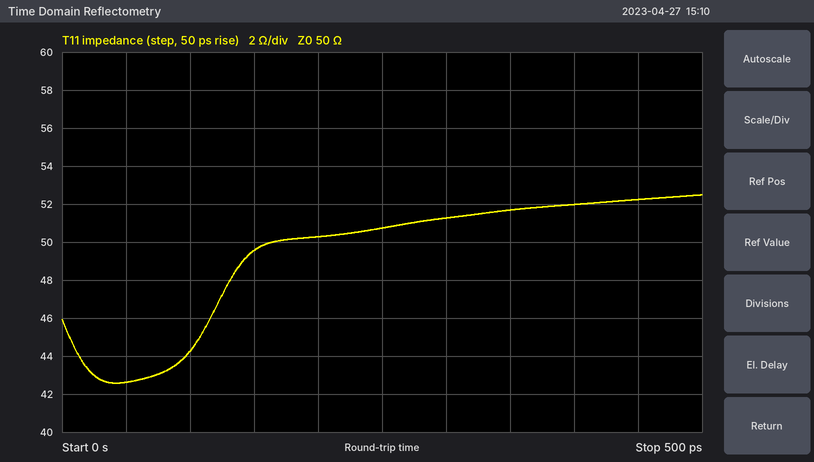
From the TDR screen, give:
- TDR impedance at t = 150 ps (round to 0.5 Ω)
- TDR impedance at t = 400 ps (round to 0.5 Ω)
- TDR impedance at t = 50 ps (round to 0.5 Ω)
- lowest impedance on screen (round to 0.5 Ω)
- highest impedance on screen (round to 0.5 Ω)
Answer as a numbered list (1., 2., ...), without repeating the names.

1. 49.5 Ω
2. 52.0 Ω
3. 42.5 Ω
4. 42.5 Ω
5. 52.5 Ω
